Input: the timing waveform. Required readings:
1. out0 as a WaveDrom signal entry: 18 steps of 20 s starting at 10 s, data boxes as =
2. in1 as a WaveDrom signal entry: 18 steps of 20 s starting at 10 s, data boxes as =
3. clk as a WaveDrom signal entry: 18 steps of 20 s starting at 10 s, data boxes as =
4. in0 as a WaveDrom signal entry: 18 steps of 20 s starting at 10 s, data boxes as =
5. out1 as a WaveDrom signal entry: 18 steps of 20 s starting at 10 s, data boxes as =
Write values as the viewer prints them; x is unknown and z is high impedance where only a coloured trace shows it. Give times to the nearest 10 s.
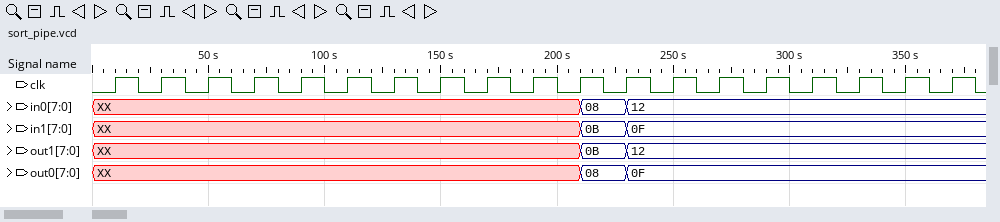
{name: 'out0', wave: 'x.........==......', data: '08 0F'}
{name: 'in1', wave: 'x.........==......', data: '0B 0F'}
{name: 'clk', wave: 'p.................'}
{name: 'in0', wave: 'x.........==......', data: '08 12'}
{name: 'out1', wave: 'x.........==......', data: '0B 12'}
